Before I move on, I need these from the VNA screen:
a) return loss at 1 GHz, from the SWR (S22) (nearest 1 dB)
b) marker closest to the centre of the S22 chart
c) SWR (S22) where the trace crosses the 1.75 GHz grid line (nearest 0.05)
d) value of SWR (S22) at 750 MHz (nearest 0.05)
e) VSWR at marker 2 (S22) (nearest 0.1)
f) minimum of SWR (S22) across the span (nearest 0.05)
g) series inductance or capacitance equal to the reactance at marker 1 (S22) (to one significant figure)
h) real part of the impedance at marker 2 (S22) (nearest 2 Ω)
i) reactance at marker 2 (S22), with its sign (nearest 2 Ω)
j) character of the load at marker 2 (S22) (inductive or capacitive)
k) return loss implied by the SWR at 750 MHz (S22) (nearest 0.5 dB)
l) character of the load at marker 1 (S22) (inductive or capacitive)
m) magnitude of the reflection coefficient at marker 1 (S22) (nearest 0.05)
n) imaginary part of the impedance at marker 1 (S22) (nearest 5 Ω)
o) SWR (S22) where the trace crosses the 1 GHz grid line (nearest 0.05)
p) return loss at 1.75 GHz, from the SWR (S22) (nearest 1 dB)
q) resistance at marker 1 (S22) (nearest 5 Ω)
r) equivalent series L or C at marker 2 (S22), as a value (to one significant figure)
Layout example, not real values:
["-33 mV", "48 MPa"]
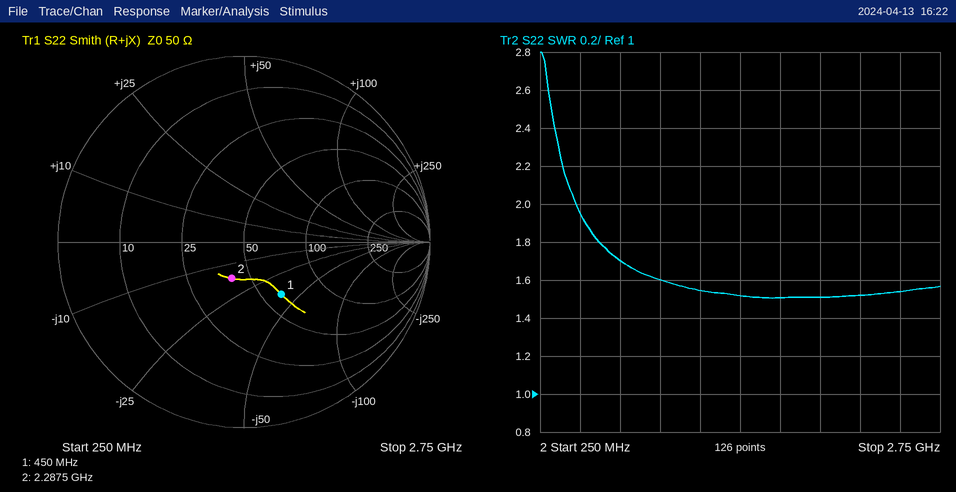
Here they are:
["13 dB", "marker 2", "1.50", "1.70", "1.5", "1.50", "9 pF", "40 Ω", "-16 Ω", "capacitive", "11.5 dB", "capacitive", "0.35", "-40 Ω", "1.60", "14 dB", "60 Ω", "4 pF"]
